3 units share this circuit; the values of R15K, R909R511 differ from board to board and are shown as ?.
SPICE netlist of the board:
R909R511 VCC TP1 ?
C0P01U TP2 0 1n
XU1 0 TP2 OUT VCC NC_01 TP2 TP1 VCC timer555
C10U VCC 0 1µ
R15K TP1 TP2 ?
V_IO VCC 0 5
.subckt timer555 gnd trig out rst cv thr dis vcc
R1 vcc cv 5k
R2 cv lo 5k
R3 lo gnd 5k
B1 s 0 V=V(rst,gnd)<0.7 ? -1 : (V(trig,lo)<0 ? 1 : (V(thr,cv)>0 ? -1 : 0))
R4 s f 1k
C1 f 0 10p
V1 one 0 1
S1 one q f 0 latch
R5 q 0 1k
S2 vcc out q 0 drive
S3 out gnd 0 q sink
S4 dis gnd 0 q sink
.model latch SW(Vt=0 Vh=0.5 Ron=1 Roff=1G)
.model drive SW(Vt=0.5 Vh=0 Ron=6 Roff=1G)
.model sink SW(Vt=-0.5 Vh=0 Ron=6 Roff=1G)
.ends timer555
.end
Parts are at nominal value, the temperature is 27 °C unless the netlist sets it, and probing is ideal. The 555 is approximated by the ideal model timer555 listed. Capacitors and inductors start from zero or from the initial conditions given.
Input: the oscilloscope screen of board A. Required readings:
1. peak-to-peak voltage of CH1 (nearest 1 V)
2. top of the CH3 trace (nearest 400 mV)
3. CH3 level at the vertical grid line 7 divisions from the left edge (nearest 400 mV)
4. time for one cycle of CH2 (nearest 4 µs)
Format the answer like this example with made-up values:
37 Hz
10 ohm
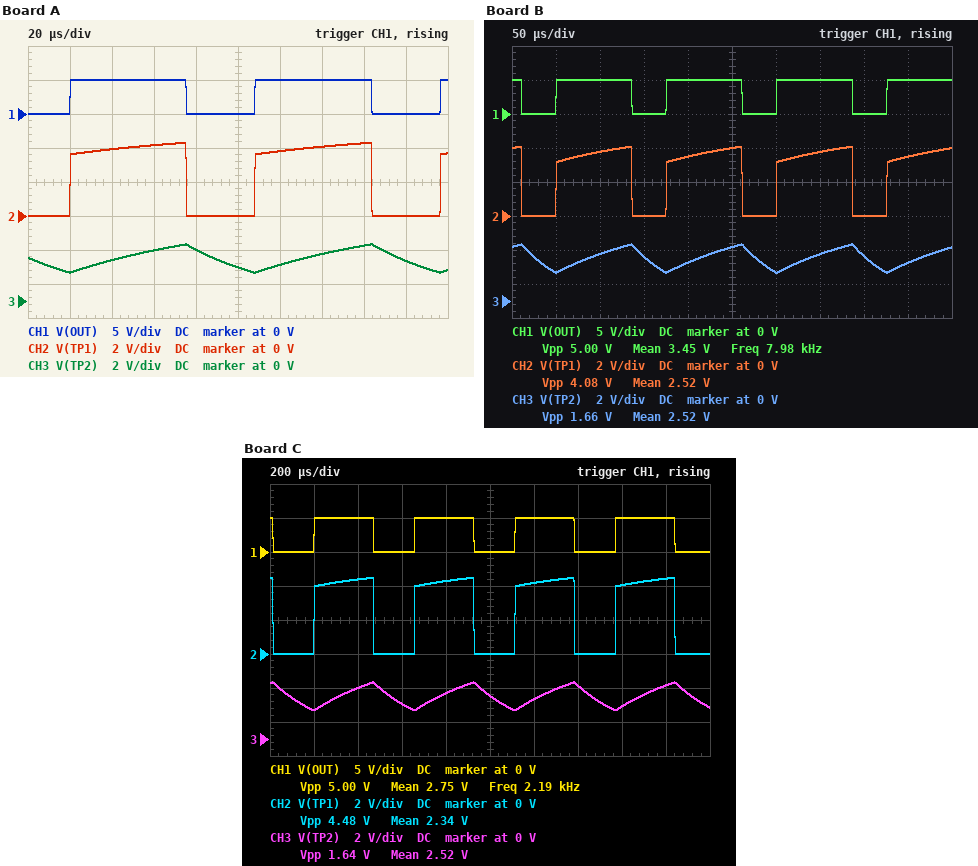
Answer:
5 V
3.2 V
2.8 V
88 µs
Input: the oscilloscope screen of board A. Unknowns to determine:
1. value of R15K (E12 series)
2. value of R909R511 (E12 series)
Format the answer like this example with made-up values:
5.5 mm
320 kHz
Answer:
47 kΩ
33 kΩ
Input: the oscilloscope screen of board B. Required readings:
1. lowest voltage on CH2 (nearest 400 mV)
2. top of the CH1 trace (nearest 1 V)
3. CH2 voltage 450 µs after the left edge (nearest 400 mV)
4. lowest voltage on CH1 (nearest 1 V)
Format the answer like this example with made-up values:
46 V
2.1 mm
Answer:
0 V
5 V
3.6 V
0 V
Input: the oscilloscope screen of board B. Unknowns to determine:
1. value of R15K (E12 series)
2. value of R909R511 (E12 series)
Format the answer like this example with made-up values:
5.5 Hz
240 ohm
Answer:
56 kΩ
68 kΩ
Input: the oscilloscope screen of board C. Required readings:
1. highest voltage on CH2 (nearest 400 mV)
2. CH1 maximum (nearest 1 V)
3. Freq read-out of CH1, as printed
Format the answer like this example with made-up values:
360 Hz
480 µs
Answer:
4.4 V
5 V
2.19 kHz
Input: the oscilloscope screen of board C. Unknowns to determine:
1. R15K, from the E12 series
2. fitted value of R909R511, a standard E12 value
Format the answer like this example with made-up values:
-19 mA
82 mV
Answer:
270 kΩ
120 kΩ
